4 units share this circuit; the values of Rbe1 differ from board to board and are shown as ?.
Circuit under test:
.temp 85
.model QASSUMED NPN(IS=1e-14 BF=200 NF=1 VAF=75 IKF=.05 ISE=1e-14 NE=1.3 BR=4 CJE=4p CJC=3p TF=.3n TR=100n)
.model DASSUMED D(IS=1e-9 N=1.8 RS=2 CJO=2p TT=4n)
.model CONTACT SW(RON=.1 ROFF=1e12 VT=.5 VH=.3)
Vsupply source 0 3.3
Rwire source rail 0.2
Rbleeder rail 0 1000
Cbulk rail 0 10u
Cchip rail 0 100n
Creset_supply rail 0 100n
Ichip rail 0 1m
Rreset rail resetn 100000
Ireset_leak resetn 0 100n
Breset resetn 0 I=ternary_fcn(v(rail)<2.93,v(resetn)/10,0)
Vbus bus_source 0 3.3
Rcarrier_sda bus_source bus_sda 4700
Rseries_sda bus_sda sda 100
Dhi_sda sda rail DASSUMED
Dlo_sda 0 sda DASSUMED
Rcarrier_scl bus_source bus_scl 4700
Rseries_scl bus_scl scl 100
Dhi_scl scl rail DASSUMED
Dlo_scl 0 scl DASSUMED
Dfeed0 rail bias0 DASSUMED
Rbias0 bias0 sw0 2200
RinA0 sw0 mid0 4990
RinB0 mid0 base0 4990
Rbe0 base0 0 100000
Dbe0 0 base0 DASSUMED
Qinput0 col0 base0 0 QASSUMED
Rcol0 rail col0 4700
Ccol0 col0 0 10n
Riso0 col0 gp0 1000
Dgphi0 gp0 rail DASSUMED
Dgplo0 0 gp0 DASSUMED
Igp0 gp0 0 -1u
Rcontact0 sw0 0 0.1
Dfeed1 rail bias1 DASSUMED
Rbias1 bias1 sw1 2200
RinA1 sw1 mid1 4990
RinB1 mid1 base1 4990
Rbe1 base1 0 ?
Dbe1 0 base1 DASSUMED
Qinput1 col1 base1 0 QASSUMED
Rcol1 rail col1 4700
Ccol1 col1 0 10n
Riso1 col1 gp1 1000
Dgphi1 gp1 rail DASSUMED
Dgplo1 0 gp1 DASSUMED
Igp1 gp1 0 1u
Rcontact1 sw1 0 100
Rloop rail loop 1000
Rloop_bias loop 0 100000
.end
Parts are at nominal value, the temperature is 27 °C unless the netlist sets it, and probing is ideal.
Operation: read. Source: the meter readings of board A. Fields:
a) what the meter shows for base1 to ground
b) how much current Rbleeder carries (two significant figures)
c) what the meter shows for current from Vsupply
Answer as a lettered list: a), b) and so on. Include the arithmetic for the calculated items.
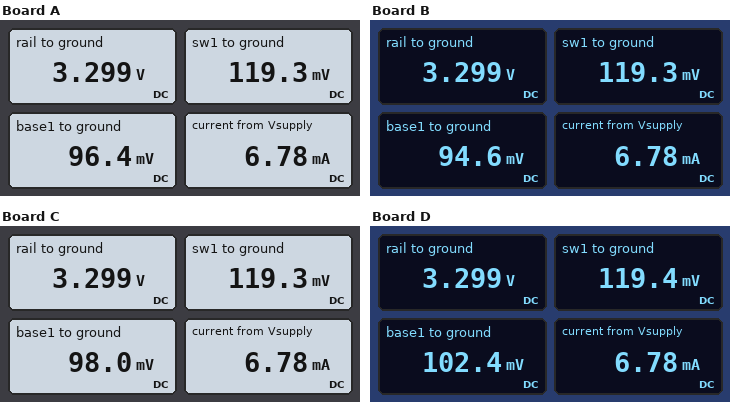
a) 96.4 mV
b) (3.299 V) / 1 kΩ = 3.3 mA
c) 6.78 mA
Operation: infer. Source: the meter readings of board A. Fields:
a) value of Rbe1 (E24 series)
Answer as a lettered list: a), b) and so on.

a) 43 kΩ
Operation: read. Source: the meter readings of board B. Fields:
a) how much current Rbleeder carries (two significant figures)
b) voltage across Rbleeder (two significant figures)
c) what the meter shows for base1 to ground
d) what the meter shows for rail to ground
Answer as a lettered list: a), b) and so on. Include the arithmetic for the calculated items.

a) (3.299 V) / 1 kΩ = 3.3 mA
b) 3.299 V = 3.3 V
c) 94.6 mV
d) 3.299 V
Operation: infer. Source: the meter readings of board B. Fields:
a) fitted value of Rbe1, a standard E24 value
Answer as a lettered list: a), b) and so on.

a) 39 kΩ
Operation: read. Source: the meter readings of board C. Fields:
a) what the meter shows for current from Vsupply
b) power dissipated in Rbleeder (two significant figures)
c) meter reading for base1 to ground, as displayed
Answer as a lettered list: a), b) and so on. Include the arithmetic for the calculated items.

a) 6.78 mA
b) (3.299 V)^2 / 1 kΩ = 11 mW
c) 98.0 mV
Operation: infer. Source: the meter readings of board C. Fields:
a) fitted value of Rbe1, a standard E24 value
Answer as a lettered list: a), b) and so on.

a) 47 kΩ
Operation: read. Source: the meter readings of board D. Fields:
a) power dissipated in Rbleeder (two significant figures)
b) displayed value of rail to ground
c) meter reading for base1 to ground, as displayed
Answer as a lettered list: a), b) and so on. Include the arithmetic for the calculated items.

a) (3.299 V)^2 / 1 kΩ = 11 mW
b) 3.299 V
c) 102.4 mV
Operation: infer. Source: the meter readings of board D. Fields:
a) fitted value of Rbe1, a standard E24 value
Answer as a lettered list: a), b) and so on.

a) 62 kΩ
